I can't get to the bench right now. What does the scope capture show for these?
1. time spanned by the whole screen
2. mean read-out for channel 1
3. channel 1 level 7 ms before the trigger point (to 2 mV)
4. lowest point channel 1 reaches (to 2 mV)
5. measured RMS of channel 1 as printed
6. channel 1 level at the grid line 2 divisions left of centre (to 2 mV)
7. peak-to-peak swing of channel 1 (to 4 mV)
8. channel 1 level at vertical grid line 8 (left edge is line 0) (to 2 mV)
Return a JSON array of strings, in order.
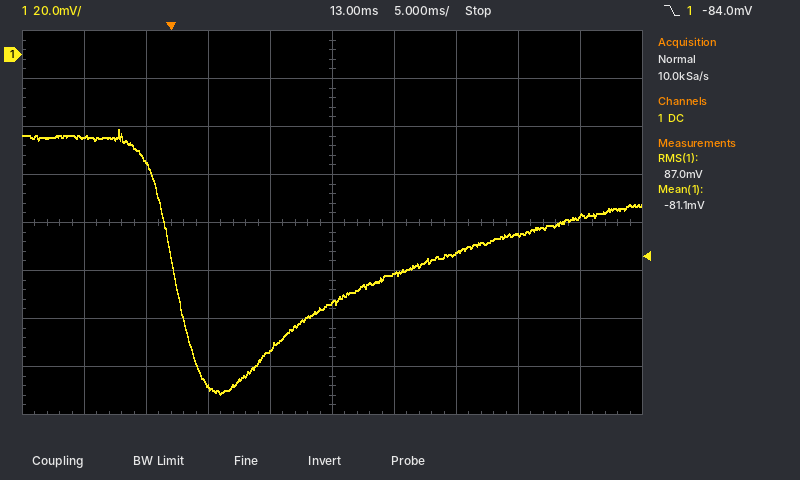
["50 ms", "-81.1 mV", "-34 mV", "-142 mV", "87.0 mV", "-138 mV", "112 mV", "-76 mV"]
